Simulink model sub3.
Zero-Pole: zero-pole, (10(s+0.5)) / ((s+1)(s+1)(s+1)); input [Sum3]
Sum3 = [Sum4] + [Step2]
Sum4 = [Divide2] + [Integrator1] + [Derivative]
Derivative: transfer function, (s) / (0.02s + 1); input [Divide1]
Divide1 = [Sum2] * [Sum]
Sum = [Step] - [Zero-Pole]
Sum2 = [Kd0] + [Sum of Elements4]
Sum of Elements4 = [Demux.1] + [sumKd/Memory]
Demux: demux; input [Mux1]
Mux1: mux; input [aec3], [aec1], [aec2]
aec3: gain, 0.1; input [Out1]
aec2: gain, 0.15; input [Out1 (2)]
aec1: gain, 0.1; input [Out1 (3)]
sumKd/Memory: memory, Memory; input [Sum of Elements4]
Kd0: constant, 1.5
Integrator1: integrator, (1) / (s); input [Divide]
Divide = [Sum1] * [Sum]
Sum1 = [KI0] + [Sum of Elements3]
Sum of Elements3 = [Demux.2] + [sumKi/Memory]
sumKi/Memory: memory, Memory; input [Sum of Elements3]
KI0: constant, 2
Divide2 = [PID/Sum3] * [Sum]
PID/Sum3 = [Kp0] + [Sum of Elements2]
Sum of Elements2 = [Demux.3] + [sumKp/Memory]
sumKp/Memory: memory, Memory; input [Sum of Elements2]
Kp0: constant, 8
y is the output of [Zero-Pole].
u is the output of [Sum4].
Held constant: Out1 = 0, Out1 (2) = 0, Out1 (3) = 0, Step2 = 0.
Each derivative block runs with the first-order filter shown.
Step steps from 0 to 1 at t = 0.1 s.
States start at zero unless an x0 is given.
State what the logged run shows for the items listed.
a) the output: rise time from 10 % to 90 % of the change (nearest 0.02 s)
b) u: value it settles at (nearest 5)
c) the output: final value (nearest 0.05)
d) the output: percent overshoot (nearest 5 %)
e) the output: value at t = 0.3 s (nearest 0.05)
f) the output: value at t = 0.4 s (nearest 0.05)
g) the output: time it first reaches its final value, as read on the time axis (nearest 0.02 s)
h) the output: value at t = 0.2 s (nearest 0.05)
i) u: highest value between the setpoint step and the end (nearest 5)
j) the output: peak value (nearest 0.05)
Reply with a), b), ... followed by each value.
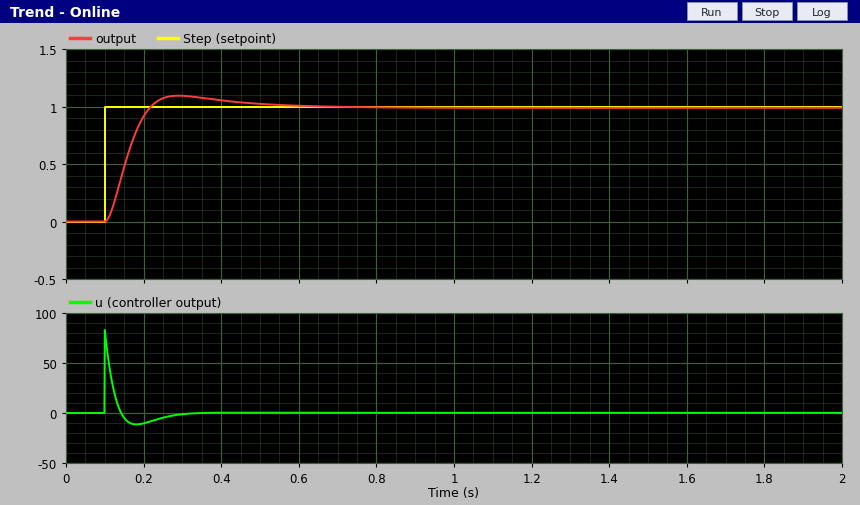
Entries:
a) 0.08 s
b) 0
c) 1.00
d) 10 %
e) 1.10
f) 1.05
g) 0.22 s
h) 0.90
i) 85
j) 1.10
